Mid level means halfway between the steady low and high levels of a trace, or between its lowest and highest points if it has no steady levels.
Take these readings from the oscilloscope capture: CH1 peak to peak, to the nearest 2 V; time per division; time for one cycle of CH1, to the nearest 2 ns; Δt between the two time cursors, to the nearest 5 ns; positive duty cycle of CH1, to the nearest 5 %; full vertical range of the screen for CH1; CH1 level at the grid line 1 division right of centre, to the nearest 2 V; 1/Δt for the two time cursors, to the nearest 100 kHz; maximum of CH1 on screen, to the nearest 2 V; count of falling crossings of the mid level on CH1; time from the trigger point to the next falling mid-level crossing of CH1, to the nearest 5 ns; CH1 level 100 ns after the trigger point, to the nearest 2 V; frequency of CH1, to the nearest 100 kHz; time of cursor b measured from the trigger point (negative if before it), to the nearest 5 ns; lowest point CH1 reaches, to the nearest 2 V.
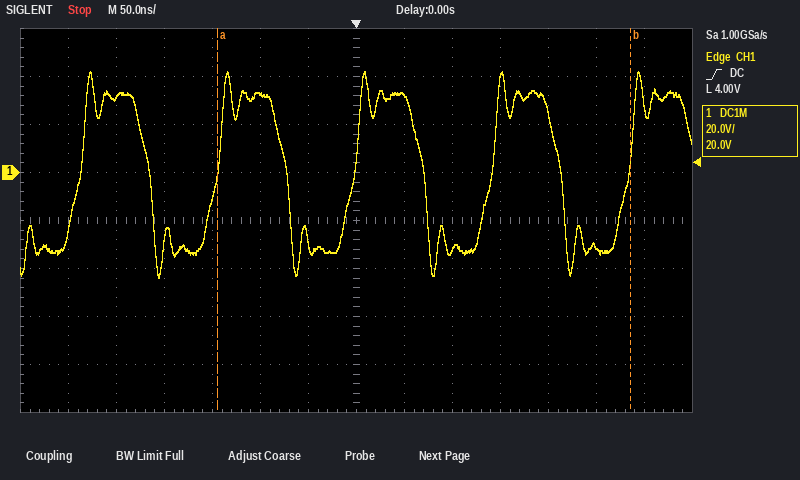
86 V
50 ns
142 ns
430 ns
50 %
160 V
32 V
2.3 MHz
42 V
4
70 ns
-32 V
7.0 MHz
+285 ns
-44 V
